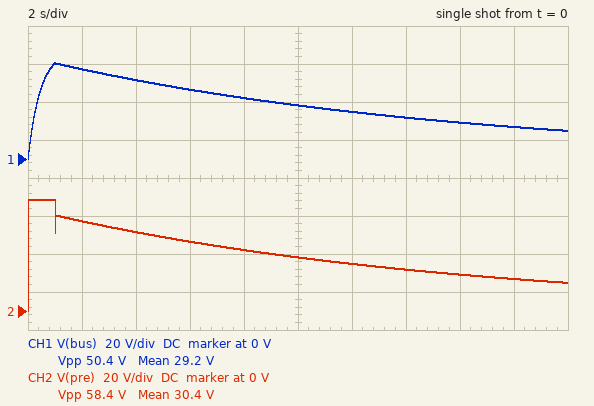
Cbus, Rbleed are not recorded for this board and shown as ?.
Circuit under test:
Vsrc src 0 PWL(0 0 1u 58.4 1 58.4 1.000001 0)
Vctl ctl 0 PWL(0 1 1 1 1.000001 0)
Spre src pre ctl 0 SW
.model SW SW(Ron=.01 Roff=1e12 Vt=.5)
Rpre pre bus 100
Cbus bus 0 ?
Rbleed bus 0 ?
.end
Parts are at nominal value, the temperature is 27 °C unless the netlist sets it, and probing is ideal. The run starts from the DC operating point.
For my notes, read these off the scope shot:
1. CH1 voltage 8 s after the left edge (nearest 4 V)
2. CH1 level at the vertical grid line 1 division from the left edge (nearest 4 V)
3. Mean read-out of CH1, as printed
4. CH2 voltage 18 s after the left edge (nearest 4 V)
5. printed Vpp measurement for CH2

32 V
48 V
29.2 V
16 V
58.4 V
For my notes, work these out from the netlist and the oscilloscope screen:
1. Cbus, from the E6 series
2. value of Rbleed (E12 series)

4.7 mF
3.3 kΩ
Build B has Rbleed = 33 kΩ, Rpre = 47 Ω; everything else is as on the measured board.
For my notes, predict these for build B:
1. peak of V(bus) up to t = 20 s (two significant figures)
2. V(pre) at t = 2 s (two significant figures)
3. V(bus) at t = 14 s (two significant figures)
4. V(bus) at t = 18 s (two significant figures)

58 V
57 V
53 V
52 V
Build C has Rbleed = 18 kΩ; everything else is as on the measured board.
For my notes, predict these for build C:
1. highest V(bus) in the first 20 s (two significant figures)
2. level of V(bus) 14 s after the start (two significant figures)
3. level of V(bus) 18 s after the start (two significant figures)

51 V
44 V
42 V
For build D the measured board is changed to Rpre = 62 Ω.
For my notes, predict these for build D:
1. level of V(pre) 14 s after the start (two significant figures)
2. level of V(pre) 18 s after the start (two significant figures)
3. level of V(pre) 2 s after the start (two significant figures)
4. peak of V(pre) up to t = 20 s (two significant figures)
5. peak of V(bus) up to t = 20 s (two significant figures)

24 V
19 V
52 V
58 V
56 V
